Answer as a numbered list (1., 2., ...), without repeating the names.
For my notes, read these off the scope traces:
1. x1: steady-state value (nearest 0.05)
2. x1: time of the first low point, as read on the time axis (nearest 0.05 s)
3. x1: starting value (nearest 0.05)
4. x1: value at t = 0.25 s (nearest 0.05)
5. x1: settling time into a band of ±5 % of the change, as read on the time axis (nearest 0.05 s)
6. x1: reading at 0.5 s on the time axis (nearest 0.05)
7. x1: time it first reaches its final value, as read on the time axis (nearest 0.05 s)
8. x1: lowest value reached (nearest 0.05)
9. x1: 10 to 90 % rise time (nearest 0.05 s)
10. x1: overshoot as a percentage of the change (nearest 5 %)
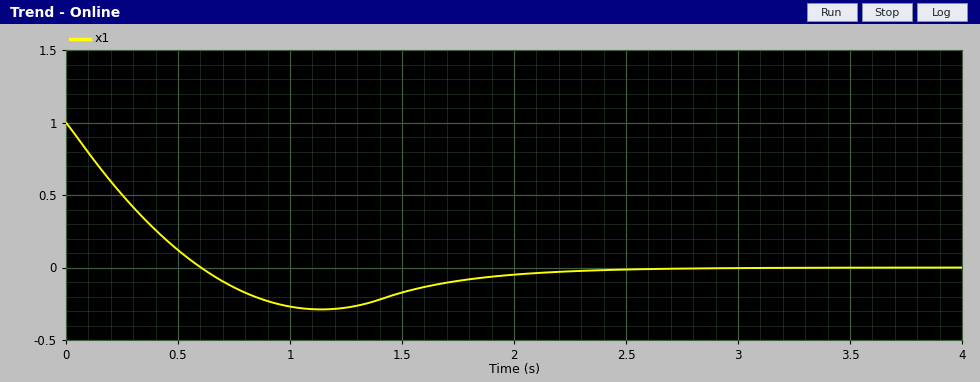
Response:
1. 0.00
2. 1.15 s
3. 1.00
4. 0.50
5. 2.00 s
6. 0.10
7. 0.60 s
8. -0.30
9. 0.45 s
10. 30 %
